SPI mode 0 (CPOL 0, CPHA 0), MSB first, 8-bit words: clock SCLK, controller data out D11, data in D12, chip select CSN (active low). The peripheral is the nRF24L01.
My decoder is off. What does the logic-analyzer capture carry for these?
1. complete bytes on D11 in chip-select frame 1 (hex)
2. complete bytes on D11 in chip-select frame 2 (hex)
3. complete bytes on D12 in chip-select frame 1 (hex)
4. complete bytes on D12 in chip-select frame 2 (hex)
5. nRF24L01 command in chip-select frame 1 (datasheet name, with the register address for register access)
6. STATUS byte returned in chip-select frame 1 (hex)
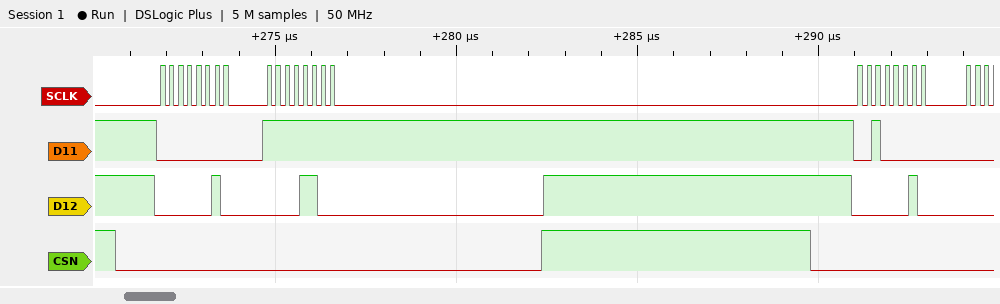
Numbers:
00 FF
20
02 0C
02
R_REGISTER 0x00
0x02
